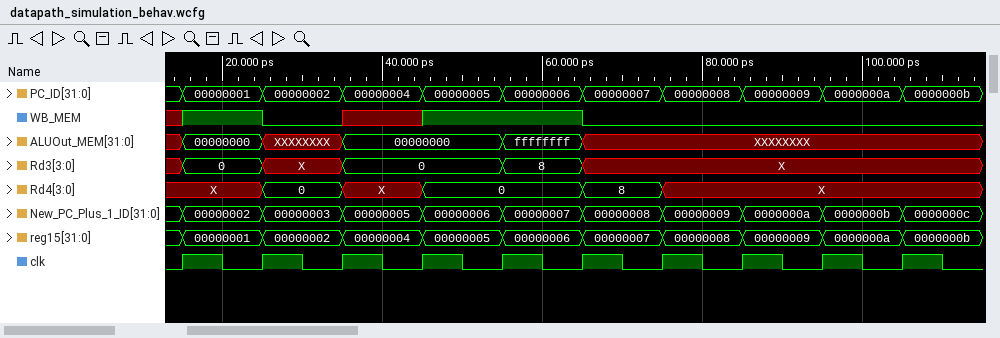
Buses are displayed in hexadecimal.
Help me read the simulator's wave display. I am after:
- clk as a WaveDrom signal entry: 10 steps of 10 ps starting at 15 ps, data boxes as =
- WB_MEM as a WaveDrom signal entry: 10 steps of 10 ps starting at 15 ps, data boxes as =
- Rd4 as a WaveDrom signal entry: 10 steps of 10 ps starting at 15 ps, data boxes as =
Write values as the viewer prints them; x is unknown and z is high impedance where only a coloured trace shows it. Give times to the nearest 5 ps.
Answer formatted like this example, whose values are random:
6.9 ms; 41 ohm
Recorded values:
{name: 'clk', wave: 'p.........'}; {name: 'WB_MEM', wave: '10x1.0....'}; {name: 'Rd4', wave: 'x=x=.=x...', data: '0 0 8'}
